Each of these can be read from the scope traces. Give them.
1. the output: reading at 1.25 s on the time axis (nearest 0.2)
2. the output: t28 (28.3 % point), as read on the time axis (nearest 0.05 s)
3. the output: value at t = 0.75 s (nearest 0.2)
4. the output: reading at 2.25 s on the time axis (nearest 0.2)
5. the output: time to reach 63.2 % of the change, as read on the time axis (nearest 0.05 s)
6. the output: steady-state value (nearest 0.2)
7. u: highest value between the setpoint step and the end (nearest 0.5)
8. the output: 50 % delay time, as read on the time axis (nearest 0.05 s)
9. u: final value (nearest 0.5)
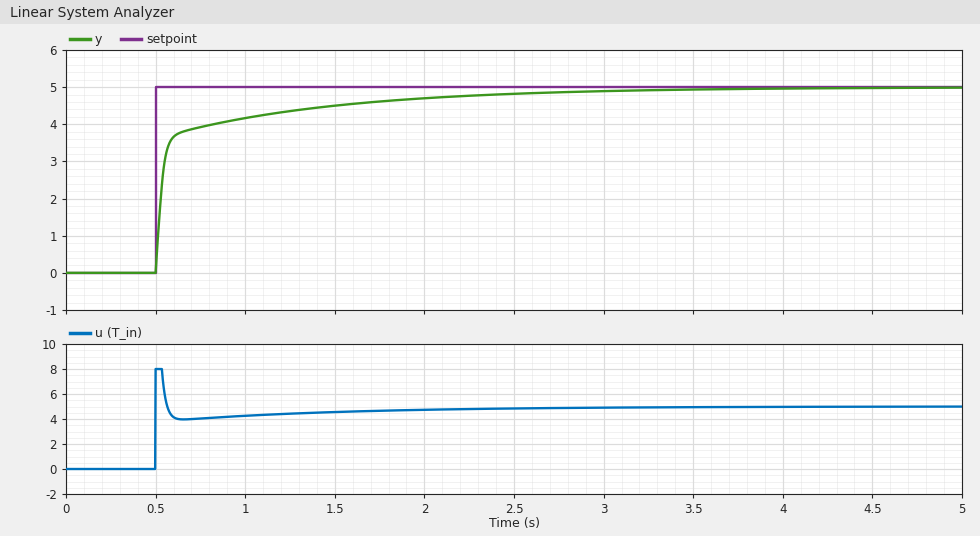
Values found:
4.4
0.50 s
4.0
4.8
0.55 s
5.0
8.0
0.55 s
5.0
